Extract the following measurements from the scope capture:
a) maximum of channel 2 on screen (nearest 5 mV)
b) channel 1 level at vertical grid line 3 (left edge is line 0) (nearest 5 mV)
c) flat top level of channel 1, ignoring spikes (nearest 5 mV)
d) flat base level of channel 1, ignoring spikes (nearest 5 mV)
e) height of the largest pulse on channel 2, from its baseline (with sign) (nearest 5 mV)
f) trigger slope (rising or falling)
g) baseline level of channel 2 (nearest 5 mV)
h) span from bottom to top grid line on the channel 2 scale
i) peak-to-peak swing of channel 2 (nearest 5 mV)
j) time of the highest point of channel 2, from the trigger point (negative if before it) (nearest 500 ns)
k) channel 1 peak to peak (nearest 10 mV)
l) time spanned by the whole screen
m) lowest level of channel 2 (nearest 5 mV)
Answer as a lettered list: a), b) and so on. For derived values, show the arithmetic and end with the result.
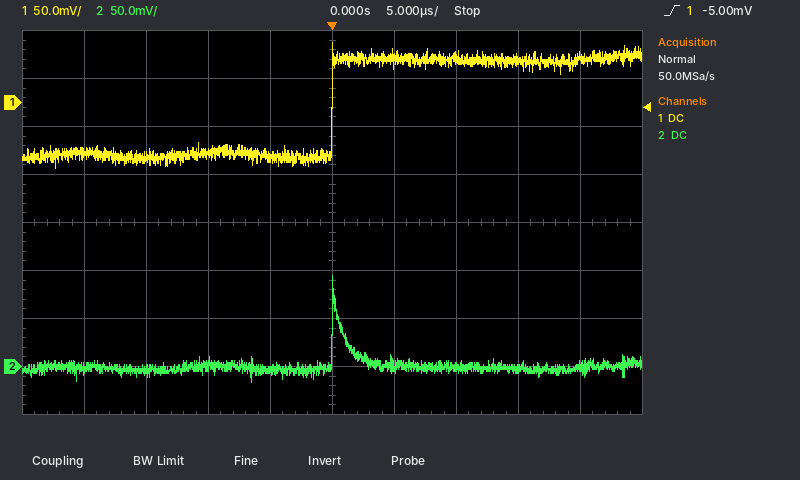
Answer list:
a) 95 mV
b) -55 mV
c) 45 mV
d) -55 mV
e) 95 mV − (0 mV) = +95 mV
f) rising
g) 0 mV
h) 400 mV
i) 95 mV − (-15 mV) = 110 mV
j) 0.0 µs
k) 130 mV
l) 50 µs
m) -15 mV
